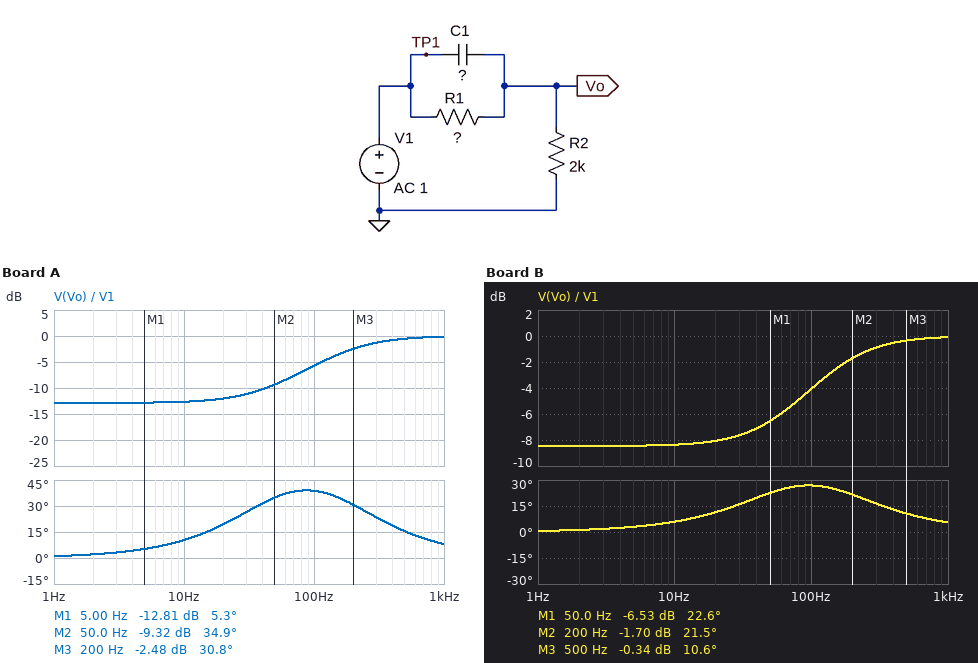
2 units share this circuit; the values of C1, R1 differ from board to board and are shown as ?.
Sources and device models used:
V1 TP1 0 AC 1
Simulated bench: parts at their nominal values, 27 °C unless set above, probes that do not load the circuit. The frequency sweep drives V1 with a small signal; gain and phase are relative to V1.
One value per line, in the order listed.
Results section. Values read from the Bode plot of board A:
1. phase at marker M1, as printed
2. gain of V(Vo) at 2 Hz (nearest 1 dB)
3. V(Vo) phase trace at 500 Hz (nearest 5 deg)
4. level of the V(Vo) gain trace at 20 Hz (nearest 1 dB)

5.3 deg
-13 dB
15 deg
-12 dB
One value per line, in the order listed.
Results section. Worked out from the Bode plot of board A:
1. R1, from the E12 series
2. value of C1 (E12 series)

6.8 kΩ
560 nF
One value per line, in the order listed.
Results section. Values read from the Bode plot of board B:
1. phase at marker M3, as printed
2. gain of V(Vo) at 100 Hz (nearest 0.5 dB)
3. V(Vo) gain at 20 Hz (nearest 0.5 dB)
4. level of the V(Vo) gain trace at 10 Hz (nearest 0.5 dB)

10.6 deg
-4.0 dB
-8.0 dB
-8.5 dB
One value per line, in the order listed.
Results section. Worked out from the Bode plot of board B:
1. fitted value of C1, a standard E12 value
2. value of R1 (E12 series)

820 nF
3.3 kΩ
